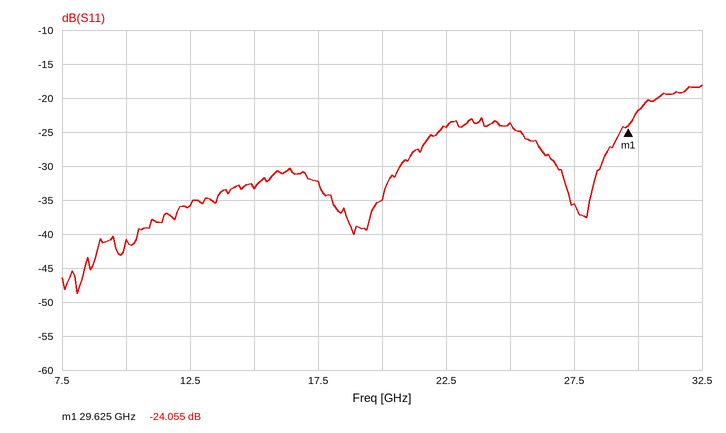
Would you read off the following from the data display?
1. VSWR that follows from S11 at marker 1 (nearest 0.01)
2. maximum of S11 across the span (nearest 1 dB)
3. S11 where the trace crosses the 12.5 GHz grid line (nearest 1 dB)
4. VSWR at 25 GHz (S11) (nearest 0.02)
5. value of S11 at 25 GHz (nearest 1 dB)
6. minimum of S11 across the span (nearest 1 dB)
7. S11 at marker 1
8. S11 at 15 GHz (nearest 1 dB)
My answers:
1.13
-18 dB
-36 dB
1.14
-24 dB
-49 dB
-24.055 dB
-33 dB
